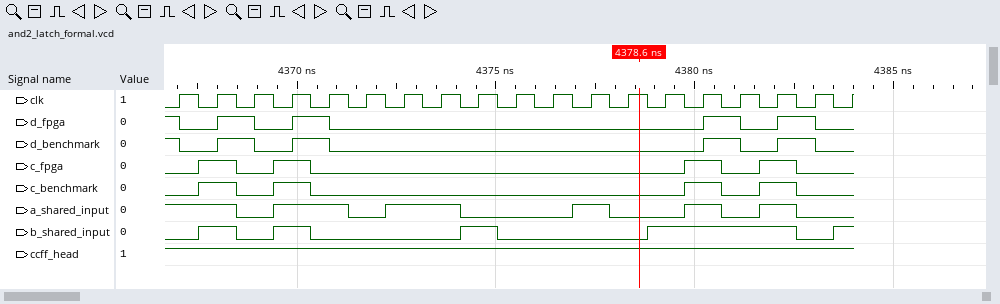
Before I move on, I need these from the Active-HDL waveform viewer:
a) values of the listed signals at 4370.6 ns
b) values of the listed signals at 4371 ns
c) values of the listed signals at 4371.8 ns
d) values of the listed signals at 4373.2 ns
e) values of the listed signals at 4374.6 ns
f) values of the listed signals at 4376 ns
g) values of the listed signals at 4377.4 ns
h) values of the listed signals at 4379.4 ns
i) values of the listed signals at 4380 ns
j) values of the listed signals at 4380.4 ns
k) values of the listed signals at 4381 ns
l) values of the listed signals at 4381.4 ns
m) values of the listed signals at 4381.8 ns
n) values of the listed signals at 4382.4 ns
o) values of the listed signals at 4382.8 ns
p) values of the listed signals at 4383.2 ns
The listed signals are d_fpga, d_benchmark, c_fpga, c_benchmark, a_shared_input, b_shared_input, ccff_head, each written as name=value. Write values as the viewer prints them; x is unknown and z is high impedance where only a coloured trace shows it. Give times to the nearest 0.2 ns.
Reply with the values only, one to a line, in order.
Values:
d_fpga=1, d_benchmark=1, c_fpga=0, c_benchmark=0, a_shared_input=1, b_shared_input=0, ccff_head=1
d_fpga=0, d_benchmark=0, c_fpga=0, c_benchmark=0, a_shared_input=1, b_shared_input=0, ccff_head=1
d_fpga=0, d_benchmark=0, c_fpga=0, c_benchmark=0, a_shared_input=0, b_shared_input=0, ccff_head=1
d_fpga=0, d_benchmark=0, c_fpga=0, c_benchmark=0, a_shared_input=1, b_shared_input=0, ccff_head=1
d_fpga=0, d_benchmark=0, c_fpga=0, c_benchmark=0, a_shared_input=0, b_shared_input=1, ccff_head=1
d_fpga=0, d_benchmark=0, c_fpga=0, c_benchmark=0, a_shared_input=0, b_shared_input=0, ccff_head=1
d_fpga=0, d_benchmark=0, c_fpga=0, c_benchmark=0, a_shared_input=1, b_shared_input=0, ccff_head=1
d_fpga=0, d_benchmark=0, c_fpga=0, c_benchmark=0, a_shared_input=0, b_shared_input=1, ccff_head=1
d_fpga=0, d_benchmark=0, c_fpga=1, c_benchmark=1, a_shared_input=1, b_shared_input=1, ccff_head=1
d_fpga=1, d_benchmark=1, c_fpga=1, c_benchmark=1, a_shared_input=1, b_shared_input=1, ccff_head=1
d_fpga=1, d_benchmark=1, c_fpga=0, c_benchmark=0, a_shared_input=0, b_shared_input=1, ccff_head=1
d_fpga=0, d_benchmark=0, c_fpga=0, c_benchmark=0, a_shared_input=0, b_shared_input=1, ccff_head=1
d_fpga=0, d_benchmark=0, c_fpga=1, c_benchmark=1, a_shared_input=1, b_shared_input=1, ccff_head=1
d_fpga=1, d_benchmark=1, c_fpga=1, c_benchmark=1, a_shared_input=1, b_shared_input=1, ccff_head=1
d_fpga=1, d_benchmark=1, c_fpga=0, c_benchmark=0, a_shared_input=0, b_shared_input=0, ccff_head=1
d_fpga=0, d_benchmark=0, c_fpga=0, c_benchmark=0, a_shared_input=0, b_shared_input=0, ccff_head=1
